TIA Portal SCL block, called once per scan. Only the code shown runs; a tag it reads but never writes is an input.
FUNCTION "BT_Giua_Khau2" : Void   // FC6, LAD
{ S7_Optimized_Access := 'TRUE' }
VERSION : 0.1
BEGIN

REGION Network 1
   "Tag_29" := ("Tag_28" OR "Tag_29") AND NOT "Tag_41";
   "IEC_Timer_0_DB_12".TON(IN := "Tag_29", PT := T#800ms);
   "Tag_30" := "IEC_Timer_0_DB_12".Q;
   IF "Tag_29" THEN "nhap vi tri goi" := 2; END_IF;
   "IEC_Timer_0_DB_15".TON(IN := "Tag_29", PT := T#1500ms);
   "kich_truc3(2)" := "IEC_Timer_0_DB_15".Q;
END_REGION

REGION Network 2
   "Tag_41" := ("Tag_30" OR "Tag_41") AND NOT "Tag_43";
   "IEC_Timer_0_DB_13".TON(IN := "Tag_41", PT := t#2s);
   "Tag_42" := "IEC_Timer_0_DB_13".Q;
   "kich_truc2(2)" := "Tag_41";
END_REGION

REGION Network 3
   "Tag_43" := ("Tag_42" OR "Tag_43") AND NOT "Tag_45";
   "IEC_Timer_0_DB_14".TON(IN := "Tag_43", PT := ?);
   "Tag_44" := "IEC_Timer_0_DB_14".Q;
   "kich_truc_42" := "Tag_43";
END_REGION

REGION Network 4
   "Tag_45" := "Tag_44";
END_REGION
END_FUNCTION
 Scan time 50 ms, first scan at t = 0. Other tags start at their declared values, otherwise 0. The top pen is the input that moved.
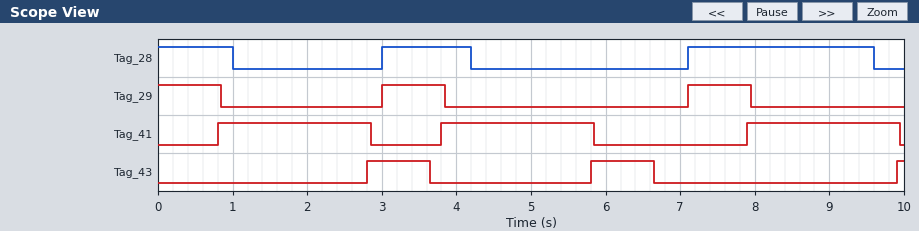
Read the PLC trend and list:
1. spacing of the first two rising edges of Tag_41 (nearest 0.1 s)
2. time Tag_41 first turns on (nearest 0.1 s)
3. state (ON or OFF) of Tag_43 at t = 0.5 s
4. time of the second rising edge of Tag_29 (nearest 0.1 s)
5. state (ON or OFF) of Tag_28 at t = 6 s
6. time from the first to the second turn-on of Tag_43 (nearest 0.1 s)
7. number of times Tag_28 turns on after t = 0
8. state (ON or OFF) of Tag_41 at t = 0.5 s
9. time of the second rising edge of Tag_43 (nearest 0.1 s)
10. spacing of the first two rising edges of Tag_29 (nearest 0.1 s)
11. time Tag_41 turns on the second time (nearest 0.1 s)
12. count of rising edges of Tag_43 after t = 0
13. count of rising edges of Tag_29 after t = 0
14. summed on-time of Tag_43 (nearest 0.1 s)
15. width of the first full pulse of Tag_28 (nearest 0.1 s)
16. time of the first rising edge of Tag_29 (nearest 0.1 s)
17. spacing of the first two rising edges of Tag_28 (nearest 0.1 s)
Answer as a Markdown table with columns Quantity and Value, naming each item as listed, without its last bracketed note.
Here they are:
| Quantity | Value |
|---|---|
| spacing of the first two rising edges of Tag_41 | 3.0 s |
| time Tag_41 first turns on | 0.8 s |
| state (ON or OFF) of Tag_43 at t = 0.5 s | OFF |
| time of the second rising edge of Tag_29 | 7.1 s |
| state (ON or OFF) of Tag_28 at t = 6 s | OFF |
| time from the first to the second turn-on of Tag_43 | 3.0 s |
| number of times Tag_28 turns on after t = 0 | 2 |
| state (ON or OFF) of Tag_41 at t = 0.5 s | OFF |
| time of the second rising edge of Tag_43 | 5.8 s |
| spacing of the first two rising edges of Tag_29 | 4.1 s |
| time Tag_41 turns on the second time | 3.8 s |
| count of rising edges of Tag_43 after t = 0 | 3 |
| count of rising edges of Tag_29 after t = 0 | 2 |
| summed on-time of Tag_43 | 1.8 s |
| width of the first full pulse of Tag_28 | 1.2 s |
| time of the first rising edge of Tag_29 | 3.0 s |
| spacing of the first two rising edges of Tag_28 | 4.1 s |
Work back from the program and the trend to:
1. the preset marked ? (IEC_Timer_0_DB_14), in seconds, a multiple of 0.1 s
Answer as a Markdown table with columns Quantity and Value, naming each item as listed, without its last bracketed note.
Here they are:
| Quantity | Value |
|---|---|
| the preset marked ? (IEC_Timer_0_DB_14), in seconds, a multiple of 0.1 s | 0.8 s |
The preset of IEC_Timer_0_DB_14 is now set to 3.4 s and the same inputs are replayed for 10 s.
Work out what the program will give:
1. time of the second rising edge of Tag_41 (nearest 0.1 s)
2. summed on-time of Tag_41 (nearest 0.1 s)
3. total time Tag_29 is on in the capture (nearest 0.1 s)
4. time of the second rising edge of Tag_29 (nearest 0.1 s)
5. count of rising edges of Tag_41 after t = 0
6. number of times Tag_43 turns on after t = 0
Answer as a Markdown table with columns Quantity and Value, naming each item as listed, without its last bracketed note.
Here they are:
| Quantity | Value |
|---|---|
| time of the second rising edge of Tag_41 | 6.3 s |
| summed on-time of Tag_41 | 4.1 s |
| total time Tag_29 is on in the capture | 5.8 s |
| time of the second rising edge of Tag_29 | 8.4 s |
| count of rising edges of Tag_41 after t = 0 | 2 |
| number of times Tag_43 turns on after t = 0 | 2 |
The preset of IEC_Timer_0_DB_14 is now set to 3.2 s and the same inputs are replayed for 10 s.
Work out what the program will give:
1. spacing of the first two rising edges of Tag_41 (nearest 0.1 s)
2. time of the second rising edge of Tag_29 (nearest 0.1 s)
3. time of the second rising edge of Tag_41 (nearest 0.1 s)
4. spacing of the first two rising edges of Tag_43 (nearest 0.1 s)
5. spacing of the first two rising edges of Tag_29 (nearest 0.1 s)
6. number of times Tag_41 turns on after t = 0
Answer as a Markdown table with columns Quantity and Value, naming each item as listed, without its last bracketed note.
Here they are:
| Quantity | Value |
|---|---|
| spacing of the first two rising edges of Tag_41 | 5.3 s |
| time of the second rising edge of Tag_29 | 8.2 s |
| time of the second rising edge of Tag_41 | 6.1 s |
| spacing of the first two rising edges of Tag_43 | 5.3 s |
| spacing of the first two rising edges of Tag_29 | 5.2 s |
| number of times Tag_41 turns on after t = 0 | 2 |
